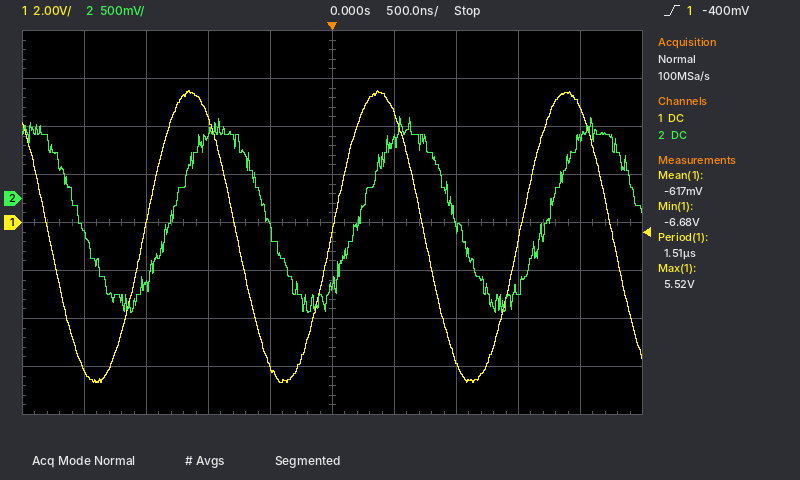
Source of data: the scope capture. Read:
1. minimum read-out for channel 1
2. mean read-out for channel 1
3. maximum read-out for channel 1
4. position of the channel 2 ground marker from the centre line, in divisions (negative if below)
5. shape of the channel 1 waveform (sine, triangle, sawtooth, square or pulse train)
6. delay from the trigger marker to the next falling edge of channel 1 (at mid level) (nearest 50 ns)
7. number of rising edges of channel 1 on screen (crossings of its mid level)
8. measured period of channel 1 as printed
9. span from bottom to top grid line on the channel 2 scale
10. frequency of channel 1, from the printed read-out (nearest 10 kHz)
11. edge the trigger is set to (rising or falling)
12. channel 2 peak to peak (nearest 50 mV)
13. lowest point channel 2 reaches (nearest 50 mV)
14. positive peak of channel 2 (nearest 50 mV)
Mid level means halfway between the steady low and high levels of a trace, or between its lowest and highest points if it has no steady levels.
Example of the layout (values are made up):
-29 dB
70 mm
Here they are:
-6.68 V
-617 mV
5.52 V
+0.5 div
sine
750 ns
3
1.51 µs
4 V
660 kHz
rising
2.05 V
-1.20 V
850 mV
